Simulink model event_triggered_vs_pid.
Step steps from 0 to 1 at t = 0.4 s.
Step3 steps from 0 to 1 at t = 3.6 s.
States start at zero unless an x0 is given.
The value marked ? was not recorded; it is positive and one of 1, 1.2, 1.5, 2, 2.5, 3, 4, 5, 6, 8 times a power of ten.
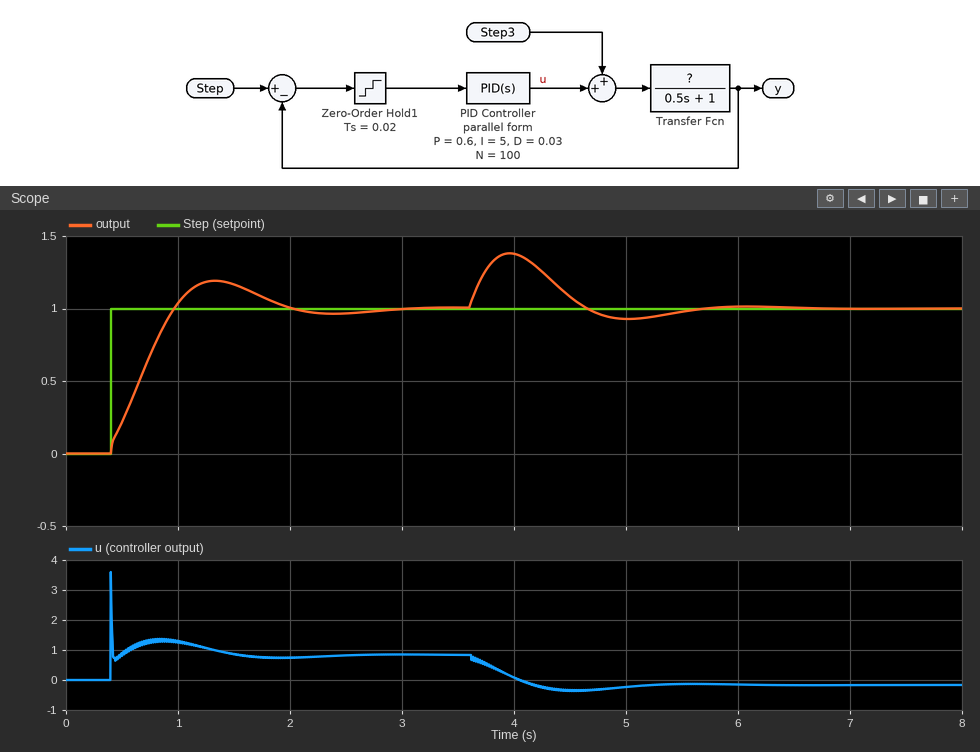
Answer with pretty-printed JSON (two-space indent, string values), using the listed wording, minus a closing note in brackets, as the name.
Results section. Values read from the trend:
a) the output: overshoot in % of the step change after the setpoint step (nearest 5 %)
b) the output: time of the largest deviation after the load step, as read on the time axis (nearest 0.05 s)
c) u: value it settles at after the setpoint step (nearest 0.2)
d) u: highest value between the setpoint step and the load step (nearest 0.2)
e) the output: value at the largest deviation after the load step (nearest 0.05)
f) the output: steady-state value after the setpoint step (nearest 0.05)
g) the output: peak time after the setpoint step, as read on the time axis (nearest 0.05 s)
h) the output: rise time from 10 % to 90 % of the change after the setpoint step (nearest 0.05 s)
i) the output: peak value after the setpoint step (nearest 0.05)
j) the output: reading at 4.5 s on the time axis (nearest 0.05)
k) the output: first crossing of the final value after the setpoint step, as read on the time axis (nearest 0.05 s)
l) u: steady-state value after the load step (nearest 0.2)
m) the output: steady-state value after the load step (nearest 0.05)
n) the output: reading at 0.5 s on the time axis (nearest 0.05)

{
  "the output: overshoot in % of the step change after the setpoint step": "20 %",
  "the output: time of the largest deviation after the load step, as read on the time axis": "3.95 s",
  "u: value it settles at after the setpoint step": "0.8",
  "u: highest value between the setpoint step and the load step": "3.6",
  "the output: value at the largest deviation after the load step": "1.40",
  "the output: steady-state value after the setpoint step": "1.00",
  "the output: peak time after the setpoint step, as read on the time axis": "1.35 s",
  "the output: rise time from 10 % to 90 % of the change after the setpoint step": "0.45 s",
  "the output: peak value after the setpoint step": "1.20",
  "the output: reading at 4.5 s on the time axis": "1.10",
  "the output: first crossing of the final value after the setpoint step, as read on the time axis": "0.95 s",
  "u: steady-state value after the load step": "-0.2",
  "the output: steady-state value after the load step": "1.00",
  "the output: reading at 0.5 s on the time axis": "0.20"
}
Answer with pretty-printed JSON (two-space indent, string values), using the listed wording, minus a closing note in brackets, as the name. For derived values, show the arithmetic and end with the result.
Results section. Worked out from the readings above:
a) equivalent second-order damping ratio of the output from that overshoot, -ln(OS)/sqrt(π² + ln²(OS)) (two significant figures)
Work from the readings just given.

{
  "equivalent second-order damping ratio of the output from that overshoot, -ln(OS)/sqrt(π² + ln²(OS))": "ln(0.2) = -1.609; 1.609 / sqrt(9.870 + 2.590) = 0.46"
}
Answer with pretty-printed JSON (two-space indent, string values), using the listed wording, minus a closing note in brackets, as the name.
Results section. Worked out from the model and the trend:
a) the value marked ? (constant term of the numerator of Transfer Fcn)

{
  "the value marked ?": "1.2"
}
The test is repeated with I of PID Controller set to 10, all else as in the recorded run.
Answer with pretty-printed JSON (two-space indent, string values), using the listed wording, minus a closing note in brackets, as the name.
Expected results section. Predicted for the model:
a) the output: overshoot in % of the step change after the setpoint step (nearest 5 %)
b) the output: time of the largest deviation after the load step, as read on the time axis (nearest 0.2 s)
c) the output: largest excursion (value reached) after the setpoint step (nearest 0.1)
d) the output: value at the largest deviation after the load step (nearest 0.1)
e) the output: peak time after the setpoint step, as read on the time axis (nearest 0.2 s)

{
  "the output: overshoot in % of the step change after the setpoint step": "35 %",
  "the output: time of the largest deviation after the load step, as read on the time axis": "3.8 s",
  "the output: largest excursion (value reached) after the setpoint step": "1.3",
  "the output: value at the largest deviation after the load step": "1.3",
  "the output: peak time after the setpoint step, as read on the time axis": "1.0 s"
}
